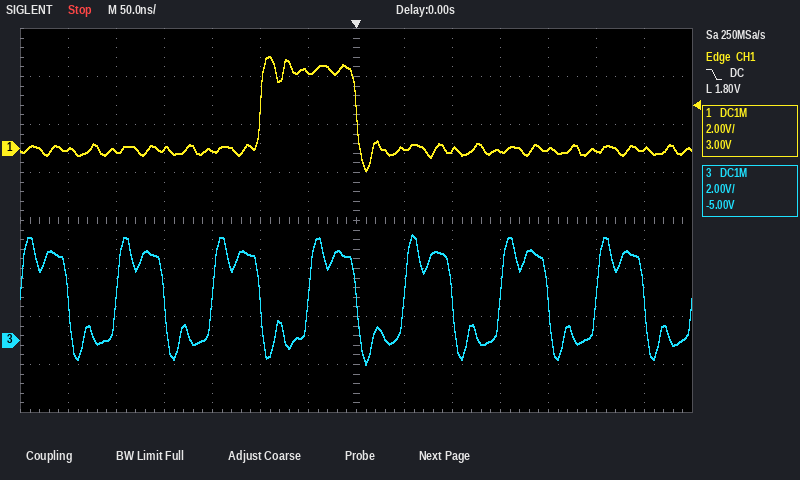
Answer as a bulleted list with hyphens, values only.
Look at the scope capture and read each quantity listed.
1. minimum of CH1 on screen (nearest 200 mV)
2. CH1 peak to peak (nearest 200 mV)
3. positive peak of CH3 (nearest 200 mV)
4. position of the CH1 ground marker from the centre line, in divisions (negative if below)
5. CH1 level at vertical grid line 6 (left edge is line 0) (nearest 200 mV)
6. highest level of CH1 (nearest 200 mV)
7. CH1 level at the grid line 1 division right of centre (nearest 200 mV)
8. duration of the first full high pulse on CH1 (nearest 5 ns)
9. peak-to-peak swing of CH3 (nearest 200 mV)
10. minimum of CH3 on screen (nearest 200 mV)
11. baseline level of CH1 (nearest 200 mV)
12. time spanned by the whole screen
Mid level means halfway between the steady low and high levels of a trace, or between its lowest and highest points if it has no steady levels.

- -1.0 V
- 4.8 V
- 4.4 V
- +1.5 div
- 3.2 V
- 3.8 V
- 0.0 V
- 100 ns
- 5.4 V
- -1.0 V
- 0.0 V
- 700 ns
